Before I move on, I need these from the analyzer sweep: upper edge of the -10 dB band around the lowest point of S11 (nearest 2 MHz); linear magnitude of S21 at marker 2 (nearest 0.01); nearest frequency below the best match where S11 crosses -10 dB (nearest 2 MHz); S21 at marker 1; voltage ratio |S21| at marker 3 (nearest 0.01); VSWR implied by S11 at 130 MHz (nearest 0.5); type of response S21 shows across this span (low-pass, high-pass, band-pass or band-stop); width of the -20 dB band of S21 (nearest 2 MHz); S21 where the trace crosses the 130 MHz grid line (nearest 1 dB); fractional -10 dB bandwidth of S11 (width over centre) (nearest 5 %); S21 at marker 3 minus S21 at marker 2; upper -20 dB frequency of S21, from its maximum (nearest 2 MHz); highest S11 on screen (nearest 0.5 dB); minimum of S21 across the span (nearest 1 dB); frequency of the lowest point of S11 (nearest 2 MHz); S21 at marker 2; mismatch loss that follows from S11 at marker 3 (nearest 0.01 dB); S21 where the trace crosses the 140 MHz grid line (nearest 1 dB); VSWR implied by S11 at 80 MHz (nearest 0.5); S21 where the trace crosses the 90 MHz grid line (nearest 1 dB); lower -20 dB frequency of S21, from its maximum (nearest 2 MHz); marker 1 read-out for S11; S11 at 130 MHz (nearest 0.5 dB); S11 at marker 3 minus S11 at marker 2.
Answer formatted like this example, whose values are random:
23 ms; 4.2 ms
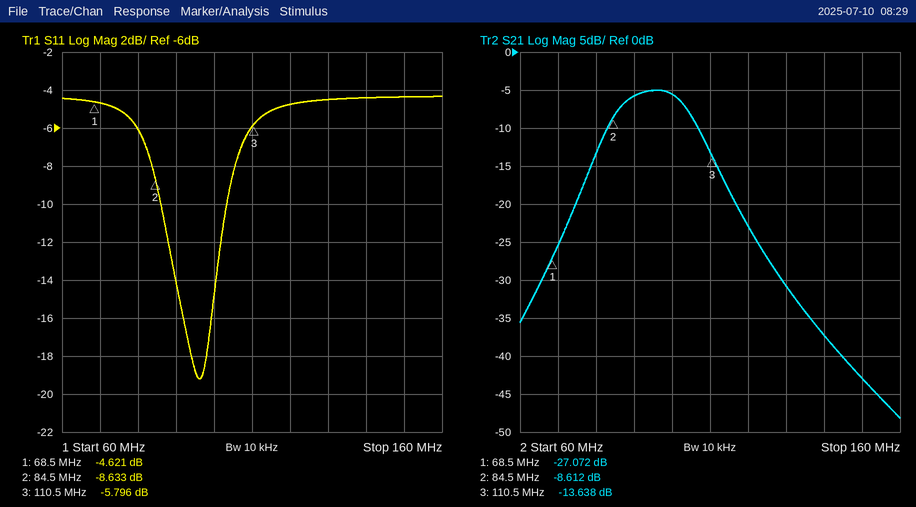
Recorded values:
104 MHz; 0.37; 86 MHz; -27.072 dB; 0.21; 4.0; band-pass; 52 MHz; -31 dB; 20 %; -5.026 dB; 122 MHz; -4.5 dB; -48 dB; 96 MHz; -8.612 dB; 1.33 dB; -37 dB; 3.0; -6 dB; 70 MHz; -4.621 dB; -4.5 dB; 2.837 dB
